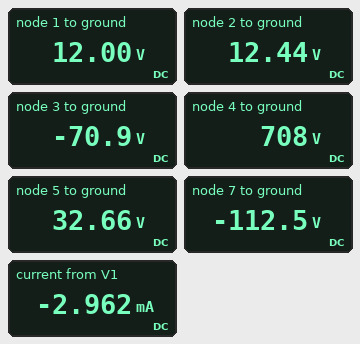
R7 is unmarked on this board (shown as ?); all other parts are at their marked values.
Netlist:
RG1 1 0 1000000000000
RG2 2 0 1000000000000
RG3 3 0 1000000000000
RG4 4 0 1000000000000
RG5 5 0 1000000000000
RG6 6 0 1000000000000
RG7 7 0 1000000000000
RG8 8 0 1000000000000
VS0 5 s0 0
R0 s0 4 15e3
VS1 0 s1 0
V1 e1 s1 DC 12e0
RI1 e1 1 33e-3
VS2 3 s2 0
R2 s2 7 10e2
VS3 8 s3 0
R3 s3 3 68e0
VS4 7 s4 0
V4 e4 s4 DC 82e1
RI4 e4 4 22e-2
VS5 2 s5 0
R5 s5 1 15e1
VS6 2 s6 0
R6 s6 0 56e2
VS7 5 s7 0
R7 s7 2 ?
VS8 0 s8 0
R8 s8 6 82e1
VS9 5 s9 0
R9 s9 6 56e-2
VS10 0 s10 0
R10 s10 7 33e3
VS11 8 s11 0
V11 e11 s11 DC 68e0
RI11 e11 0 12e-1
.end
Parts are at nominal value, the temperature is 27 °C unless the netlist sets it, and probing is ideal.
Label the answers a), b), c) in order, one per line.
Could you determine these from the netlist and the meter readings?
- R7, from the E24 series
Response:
a) 3.9 kΩ
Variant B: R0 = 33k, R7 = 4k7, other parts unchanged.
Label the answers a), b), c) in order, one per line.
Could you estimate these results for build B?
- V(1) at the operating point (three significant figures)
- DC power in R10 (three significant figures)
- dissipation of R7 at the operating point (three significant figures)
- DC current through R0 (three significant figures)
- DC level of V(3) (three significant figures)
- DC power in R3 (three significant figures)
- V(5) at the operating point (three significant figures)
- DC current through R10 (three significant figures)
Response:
a) 12.0 V
b) 236 mW
c) 5.42 mW
d) 21.7 mA
e) -69.3 V
f) 24.5 mW
g) 16.9 V
h) 2.68 mA
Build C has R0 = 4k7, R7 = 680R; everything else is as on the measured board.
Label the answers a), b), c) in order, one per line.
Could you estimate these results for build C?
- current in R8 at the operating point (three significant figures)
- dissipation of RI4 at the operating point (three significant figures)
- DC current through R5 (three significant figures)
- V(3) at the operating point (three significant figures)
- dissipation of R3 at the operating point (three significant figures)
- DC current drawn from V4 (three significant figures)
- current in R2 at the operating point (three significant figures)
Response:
a) 68.2 mA
b) 3.26 mW
c) 50.1 mA
d) -76.0 V
e) 914 mW
f) 122 mA
g) 116 mA
